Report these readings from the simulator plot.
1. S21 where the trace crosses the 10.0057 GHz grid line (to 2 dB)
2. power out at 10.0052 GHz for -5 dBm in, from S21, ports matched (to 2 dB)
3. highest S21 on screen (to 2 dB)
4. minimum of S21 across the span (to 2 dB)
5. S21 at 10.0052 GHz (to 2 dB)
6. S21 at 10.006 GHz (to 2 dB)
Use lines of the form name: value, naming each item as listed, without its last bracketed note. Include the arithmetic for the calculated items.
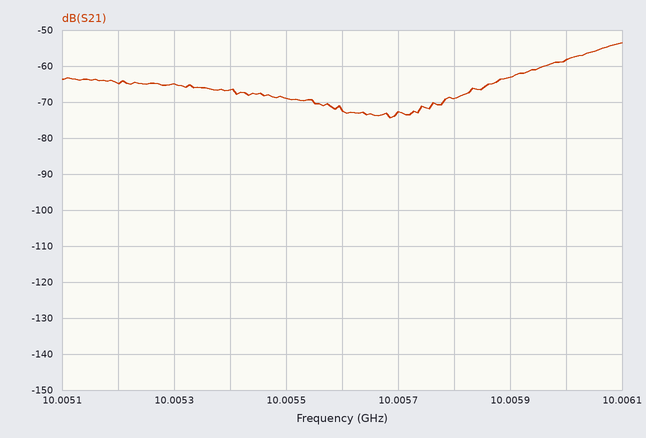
S21 where the trace crosses the 10.0057 GHz grid line: -72 dB
power out at 10.0052 GHz for -5 dBm in, from S21, ports matched: -5 dBm + (-64 dB) = -70 dBm
highest S21 on screen: -54 dB
minimum of S21 across the span: -74 dB
S21 at 10.0052 GHz: -64 dB
S21 at 10.006 GHz: -58 dB
